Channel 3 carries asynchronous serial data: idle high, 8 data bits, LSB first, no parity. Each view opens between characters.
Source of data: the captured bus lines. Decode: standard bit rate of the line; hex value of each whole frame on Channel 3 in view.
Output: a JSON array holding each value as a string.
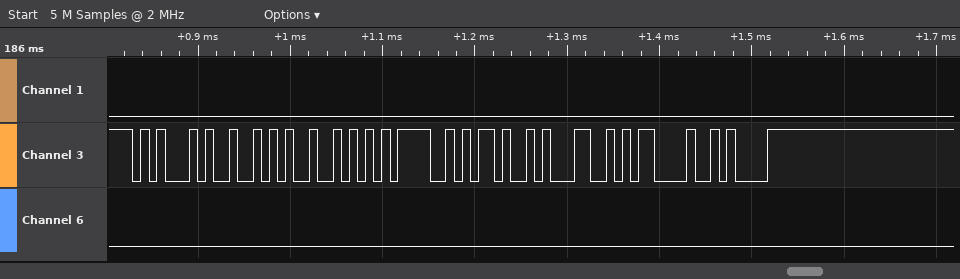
["115200 baud", "45, 52, 52, 3D, 2D, 31, 0D, 0A"]
